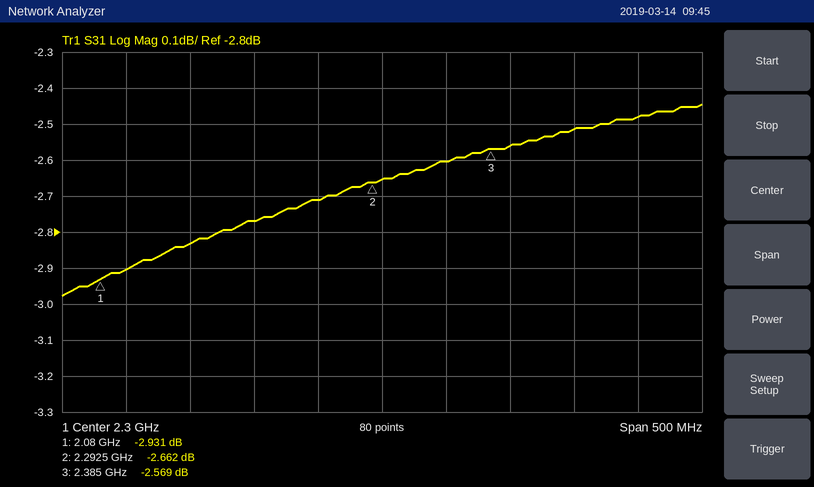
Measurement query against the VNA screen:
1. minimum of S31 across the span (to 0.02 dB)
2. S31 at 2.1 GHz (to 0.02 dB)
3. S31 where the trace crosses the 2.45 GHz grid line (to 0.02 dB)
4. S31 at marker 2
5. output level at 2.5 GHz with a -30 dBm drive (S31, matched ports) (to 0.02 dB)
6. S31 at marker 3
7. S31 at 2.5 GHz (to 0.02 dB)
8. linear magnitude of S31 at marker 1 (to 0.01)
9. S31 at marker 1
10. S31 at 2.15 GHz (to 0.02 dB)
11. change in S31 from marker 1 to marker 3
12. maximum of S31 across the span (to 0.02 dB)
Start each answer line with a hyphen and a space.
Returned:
- -2.98 dB
- -2.90 dB
- -2.52 dB
- -2.662 dB
- -32.48 dBm
- -2.569 dB
- -2.48 dB
- 0.71
- -2.931 dB
- -2.84 dB
- 0.362 dB
- -2.44 dB
